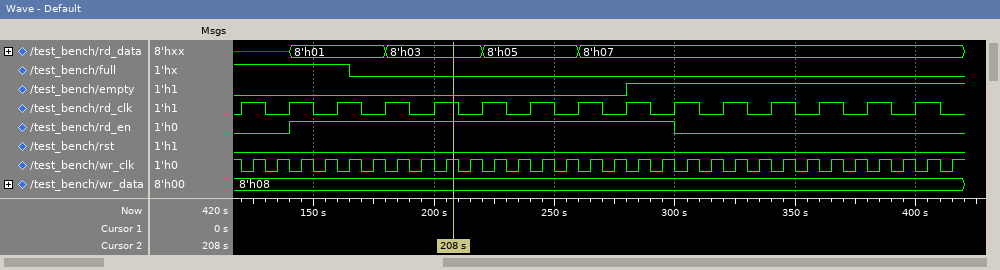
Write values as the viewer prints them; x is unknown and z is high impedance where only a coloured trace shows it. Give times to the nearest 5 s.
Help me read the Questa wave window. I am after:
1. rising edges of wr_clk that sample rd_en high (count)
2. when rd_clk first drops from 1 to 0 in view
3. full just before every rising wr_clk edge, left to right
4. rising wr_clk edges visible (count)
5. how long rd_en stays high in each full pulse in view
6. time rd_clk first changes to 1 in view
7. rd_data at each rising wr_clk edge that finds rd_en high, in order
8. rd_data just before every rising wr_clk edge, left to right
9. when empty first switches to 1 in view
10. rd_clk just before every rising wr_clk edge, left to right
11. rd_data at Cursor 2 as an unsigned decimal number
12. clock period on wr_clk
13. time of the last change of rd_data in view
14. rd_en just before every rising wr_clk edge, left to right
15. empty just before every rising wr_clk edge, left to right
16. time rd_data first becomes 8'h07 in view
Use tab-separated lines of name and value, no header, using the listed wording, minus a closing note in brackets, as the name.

rising edges of wr_clk that sample rd_en high	16
when rd_clk first drops from 1 to 0 in view	130 s
full just before every rising wr_clk edge, left to right	1 1 1 1 1 0 0 0 0 0 0 0 0 0 0 0 0 0 0 0 0 0 0 0 0 0 0 0 0 0
rising wr_clk edges visible	30
how long rd_en stays high in each full pulse in view	160 s
time rd_clk first changes to 1 in view	120 s
rd_data at each rising wr_clk edge that finds rd_en high, in order	8'h01, 8'h01, 8'h01, 8'h01, 8'h03, 8'h03, 8'h03, 8'h03, 8'h05, 8'h05, 8'h05, 8'h05, 8'h07, 8'h07, 8'h07, 8'h07
rd_data just before every rising wr_clk edge, left to right	x, x, 8'h01, 8'h01, 8'h01, 8'h01, 8'h03, 8'h03, 8'h03, 8'h03, 8'h05, 8'h05, 8'h05, 8'h05, 8'h07, 8'h07, 8'h07, 8'h07, 8'h07, 8'h07, 8'h07, 8'h07, 8'h07, 8'h07, 8'h07, 8'h07, 8'h07, 8'h07, 8'h07, 8'h07
when empty first switches to 1 in view	280 s
rd_clk just before every rising wr_clk edge, left to right	1 0 1 0 1 0 1 0 1 0 1 0 1 0 1 0 1 0 1 0 1 0 1 0 1 0 1 0 1 0
rd_data at Cursor 2 as an unsigned decimal number	3
clock period on wr_clk	10 s
time of the last change of rd_data in view	260 s
rd_en just before every rising wr_clk edge, left to right	0 0 1 1 1 1 1 1 1 1 1 1 1 1 1 1 1 1 0 0 0 0 0 0 0 0 0 0 0 0
empty just before every rising wr_clk edge, left to right	0 0 0 0 0 0 0 0 0 0 0 0 0 0 0 0 1 1 1 1 1 1 1 1 1 1 1 1 1 1
time rd_data first becomes 8'h07 in view	260 s
